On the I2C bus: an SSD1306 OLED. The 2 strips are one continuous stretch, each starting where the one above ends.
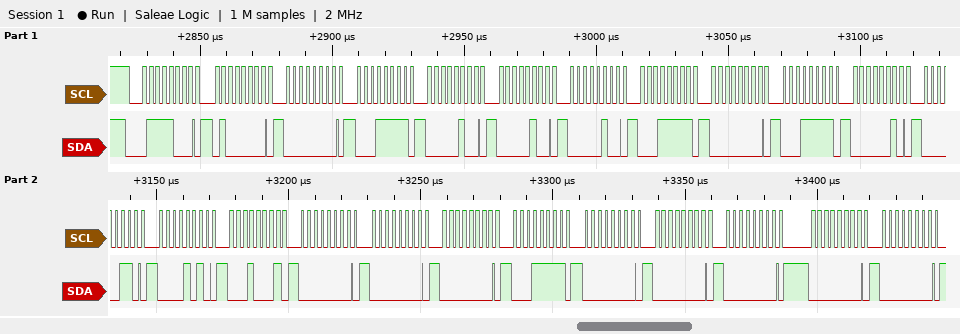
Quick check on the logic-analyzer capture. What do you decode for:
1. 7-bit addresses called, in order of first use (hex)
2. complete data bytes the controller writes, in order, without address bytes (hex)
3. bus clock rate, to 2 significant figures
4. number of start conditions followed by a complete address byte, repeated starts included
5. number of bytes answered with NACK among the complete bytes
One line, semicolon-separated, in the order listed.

0x3C; 40 00 1F 04 04 04 1F 00 1F 02 06 0A 11 00 00 00 1F 00 00 00 00 00; 400 kHz; 1; 0
